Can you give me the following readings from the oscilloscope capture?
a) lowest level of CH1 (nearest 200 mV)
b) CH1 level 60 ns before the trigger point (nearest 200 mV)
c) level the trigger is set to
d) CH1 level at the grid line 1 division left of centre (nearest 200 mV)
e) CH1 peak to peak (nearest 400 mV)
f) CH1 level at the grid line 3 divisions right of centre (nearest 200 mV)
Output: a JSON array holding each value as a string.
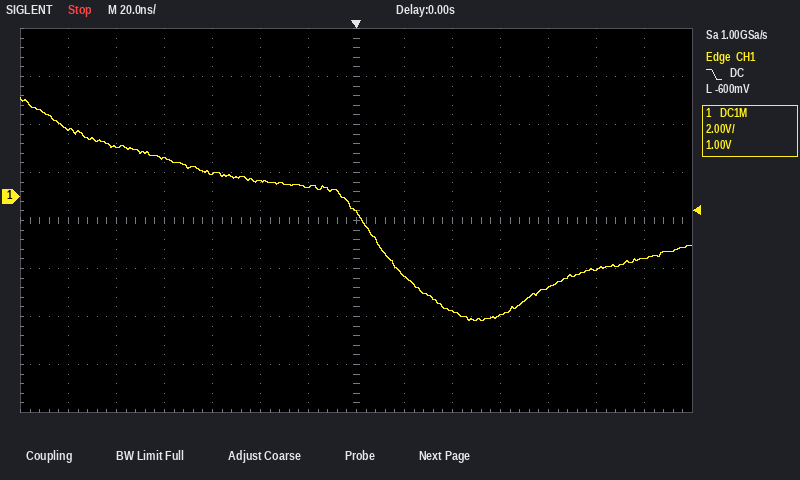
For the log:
["-5.2 V", "1.0 V", "-600 mV", "400 mV", "9.2 V", "-5.0 V"]
